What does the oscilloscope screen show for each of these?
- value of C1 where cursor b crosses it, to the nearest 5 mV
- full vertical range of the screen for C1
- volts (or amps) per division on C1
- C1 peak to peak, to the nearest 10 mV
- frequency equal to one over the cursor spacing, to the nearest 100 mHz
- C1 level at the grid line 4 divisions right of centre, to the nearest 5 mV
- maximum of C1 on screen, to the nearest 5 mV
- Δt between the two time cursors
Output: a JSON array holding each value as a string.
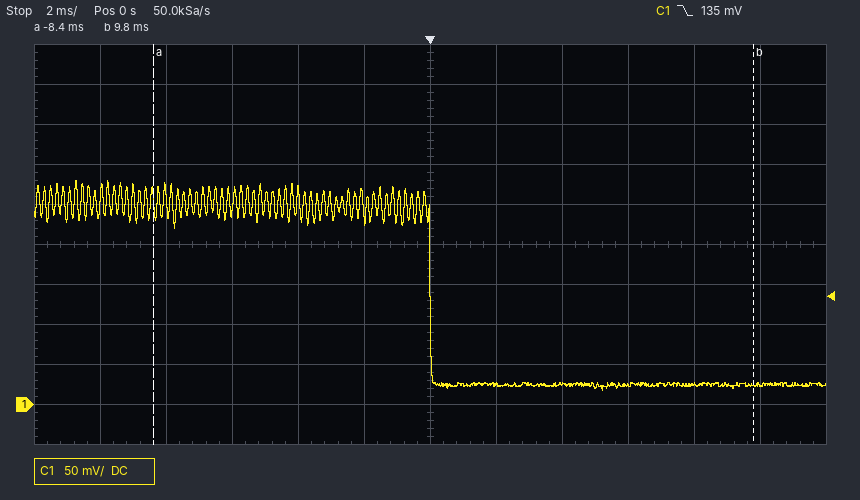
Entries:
["25 mV", "500 mV", "50 mV", "260 mV", "54.9 Hz", "25 mV", "280 mV", "18.2 ms"]
